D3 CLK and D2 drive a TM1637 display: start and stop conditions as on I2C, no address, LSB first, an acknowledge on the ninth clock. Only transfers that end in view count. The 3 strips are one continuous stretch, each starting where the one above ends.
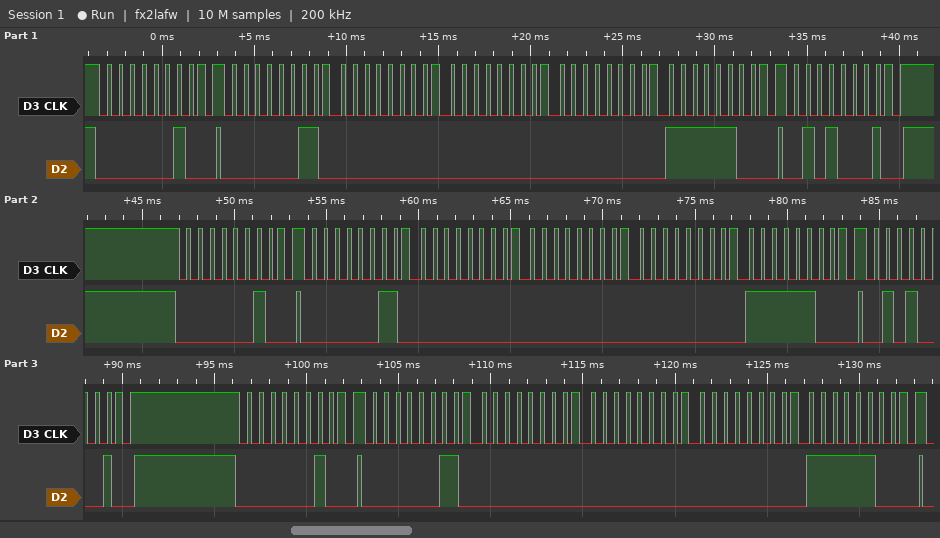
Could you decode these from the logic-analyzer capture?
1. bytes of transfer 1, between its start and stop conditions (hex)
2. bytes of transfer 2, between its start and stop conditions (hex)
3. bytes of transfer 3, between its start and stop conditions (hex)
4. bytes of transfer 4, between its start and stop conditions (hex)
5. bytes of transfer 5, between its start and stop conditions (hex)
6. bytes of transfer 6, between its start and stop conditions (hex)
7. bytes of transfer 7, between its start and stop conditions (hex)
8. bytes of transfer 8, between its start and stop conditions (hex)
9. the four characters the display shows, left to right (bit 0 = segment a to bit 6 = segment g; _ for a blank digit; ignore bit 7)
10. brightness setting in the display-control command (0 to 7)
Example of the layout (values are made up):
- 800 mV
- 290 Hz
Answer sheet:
- 40
- C0 00 00 00 3F
- 8A
- 40
- C0 00 00 00 3F
- 8A
- 40
- C0 00 00 00 3F
- ___0
- 2
